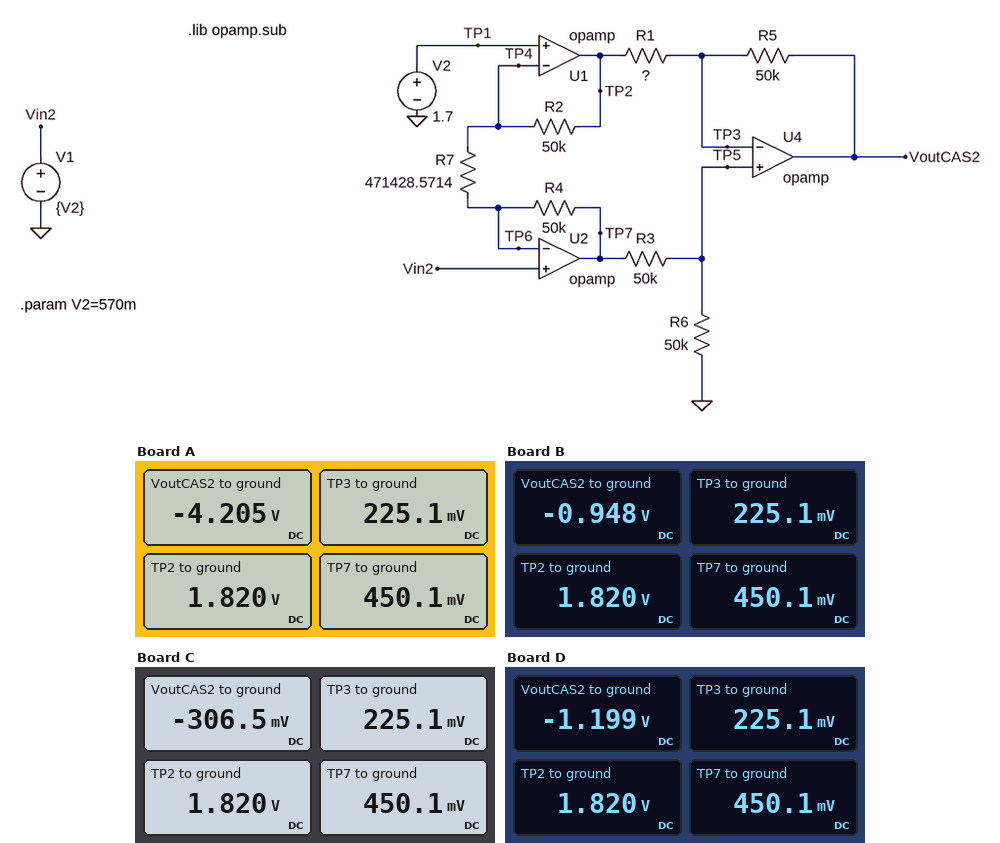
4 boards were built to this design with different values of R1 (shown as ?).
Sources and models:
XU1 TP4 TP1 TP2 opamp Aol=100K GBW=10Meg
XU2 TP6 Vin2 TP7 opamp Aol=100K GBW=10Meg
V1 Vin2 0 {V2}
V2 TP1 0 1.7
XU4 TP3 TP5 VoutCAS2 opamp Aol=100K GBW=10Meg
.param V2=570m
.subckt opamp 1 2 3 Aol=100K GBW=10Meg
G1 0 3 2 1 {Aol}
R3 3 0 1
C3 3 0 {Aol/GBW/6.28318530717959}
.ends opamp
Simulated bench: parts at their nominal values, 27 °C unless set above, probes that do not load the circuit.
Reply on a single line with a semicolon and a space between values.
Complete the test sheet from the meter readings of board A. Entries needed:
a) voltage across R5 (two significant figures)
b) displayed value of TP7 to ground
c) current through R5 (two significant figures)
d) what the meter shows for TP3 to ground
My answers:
4.4 V; 450.1 mV; 89 µA; 225.1 mV
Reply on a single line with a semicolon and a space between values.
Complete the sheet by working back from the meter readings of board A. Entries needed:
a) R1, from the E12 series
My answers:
18 kΩ
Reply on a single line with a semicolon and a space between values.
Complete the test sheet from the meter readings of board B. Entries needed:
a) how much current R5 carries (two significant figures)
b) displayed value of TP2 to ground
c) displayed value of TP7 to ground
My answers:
23 µA; 1.820 V; 450.1 mV
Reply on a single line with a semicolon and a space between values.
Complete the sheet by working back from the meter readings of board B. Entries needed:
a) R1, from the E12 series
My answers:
68 kΩ
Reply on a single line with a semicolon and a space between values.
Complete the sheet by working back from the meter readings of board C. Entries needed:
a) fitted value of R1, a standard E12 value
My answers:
150 kΩ
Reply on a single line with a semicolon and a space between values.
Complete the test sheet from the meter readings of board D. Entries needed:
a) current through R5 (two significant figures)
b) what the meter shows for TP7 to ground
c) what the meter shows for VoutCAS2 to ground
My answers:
28 µA; 450.1 mV; -1.199 V
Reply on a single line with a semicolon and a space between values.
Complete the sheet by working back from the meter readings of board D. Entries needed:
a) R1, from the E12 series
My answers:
56 kΩ
